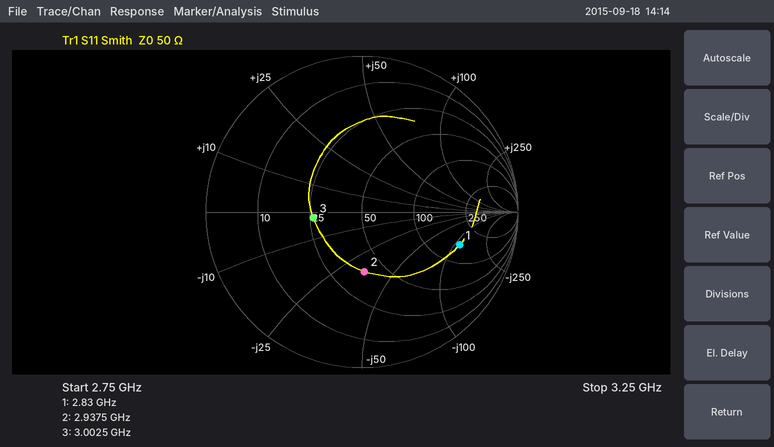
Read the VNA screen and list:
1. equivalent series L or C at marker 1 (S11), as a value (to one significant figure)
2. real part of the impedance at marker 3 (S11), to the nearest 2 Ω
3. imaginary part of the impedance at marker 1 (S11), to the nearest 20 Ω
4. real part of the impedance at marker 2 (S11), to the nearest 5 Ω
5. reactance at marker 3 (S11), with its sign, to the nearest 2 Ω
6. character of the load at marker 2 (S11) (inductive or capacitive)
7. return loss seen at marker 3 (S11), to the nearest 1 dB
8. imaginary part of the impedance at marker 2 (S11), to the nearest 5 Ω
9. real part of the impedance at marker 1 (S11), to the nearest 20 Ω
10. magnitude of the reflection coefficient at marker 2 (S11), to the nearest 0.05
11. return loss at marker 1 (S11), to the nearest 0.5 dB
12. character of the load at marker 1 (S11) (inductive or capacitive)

500 fF
26 Ω
-120 Ω
40 Ω
-2 Ω
capacitive
10 dB
-35 Ω
160 Ω
0.40
3.5 dB
capacitive
